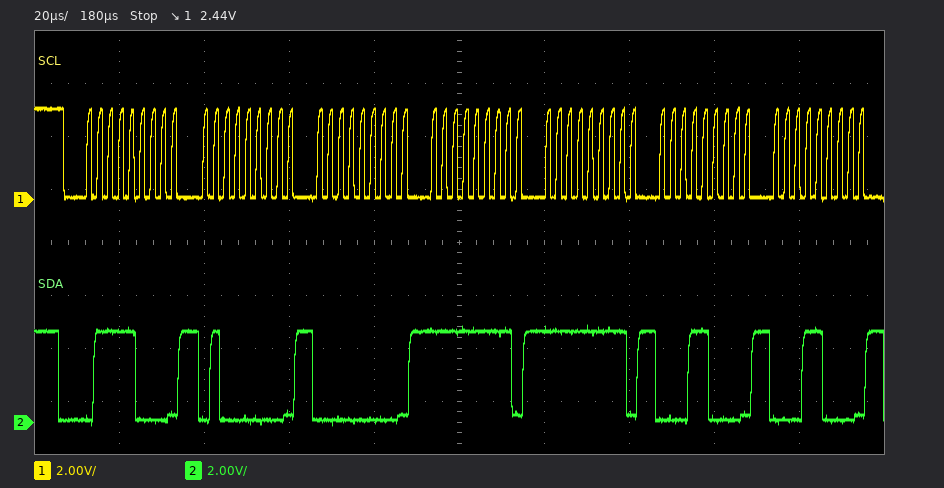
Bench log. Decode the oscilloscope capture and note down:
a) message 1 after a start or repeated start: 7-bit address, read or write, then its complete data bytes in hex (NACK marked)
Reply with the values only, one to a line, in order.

0x3C write: 40 00 FF FF 18 18
